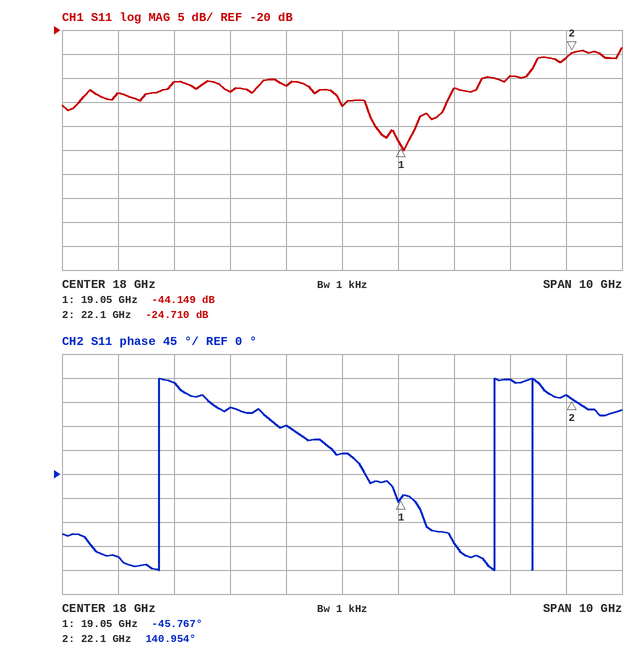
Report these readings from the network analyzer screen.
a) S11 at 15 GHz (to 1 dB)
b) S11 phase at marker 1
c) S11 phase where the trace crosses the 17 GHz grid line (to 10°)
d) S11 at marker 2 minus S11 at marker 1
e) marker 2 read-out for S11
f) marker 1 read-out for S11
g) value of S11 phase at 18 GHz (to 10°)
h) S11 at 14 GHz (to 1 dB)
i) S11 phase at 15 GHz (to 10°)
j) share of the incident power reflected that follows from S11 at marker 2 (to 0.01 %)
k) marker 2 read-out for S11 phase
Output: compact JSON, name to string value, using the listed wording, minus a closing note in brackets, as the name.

{"S11 at 15 GHz": "-31 dB", "S11 phase at marker 1": "-45.767°", "S11 phase where the trace crosses the 17 GHz grid line": "90°", "S11 at marker 2 minus S11 at marker 1": "19.439 dB", "marker 2 read-out for S11": "-24.710 dB", "marker 1 read-out for S11": "-44.149 dB", "value of S11 phase at 18 GHz": "40°", "S11 at 14 GHz": "-33 dB", "S11 phase at 15 GHz": "170°", "share of the incident power reflected that follows from S11 at marker 2": "0.34 %", "marker 2 read-out for S11 phase": "140.954°"}
